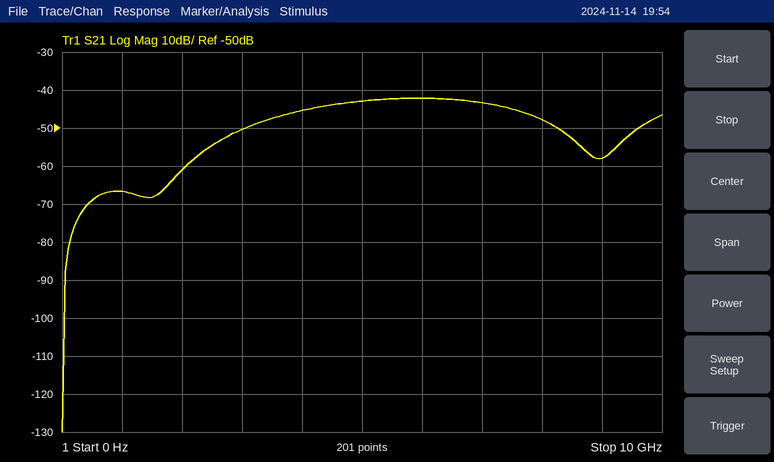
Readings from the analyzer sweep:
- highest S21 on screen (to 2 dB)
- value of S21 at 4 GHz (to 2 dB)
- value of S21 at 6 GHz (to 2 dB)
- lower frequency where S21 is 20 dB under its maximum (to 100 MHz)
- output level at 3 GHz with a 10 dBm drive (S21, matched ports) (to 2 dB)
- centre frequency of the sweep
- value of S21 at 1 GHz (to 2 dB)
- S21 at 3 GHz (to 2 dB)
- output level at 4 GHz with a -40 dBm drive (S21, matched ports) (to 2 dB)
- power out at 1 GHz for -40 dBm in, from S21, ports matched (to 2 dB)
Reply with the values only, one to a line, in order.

-42 dB
-46 dB
-42 dB
1.9 GHz
-40 dBm
5 GHz
-66 dB
-50 dB
-86 dBm
-106 dBm
